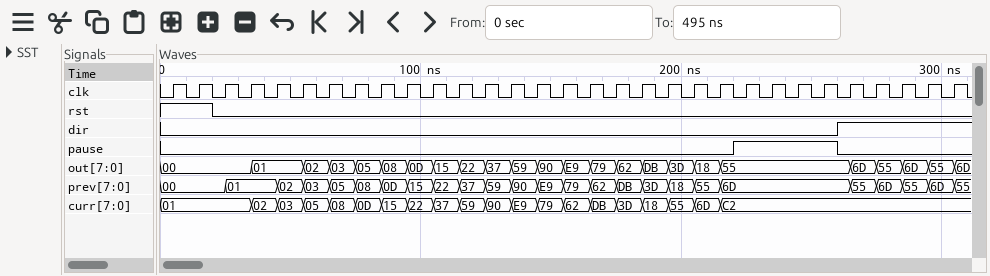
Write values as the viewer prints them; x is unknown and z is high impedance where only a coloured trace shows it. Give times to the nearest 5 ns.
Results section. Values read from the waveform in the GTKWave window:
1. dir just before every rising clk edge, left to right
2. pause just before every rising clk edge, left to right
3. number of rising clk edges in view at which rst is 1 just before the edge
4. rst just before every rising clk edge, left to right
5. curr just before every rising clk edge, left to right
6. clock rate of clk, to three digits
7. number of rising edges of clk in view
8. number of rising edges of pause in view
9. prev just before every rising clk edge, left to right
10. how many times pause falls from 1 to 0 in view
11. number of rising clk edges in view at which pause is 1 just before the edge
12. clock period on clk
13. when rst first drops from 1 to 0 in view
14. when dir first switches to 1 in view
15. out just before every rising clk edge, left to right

0 0 0 0 0 0 0 0 0 0 0 0 0 0 0 0 0 0 0 0 0 0 0 0 0 0 1 1 1 1 1
0 0 0 0 0 0 0 0 0 0 0 0 0 0 0 0 0 0 0 0 0 0 1 1 1 1 0 0 0 0 0
2
1 1 0 0 0 0 0 0 0 0 0 0 0 0 0 0 0 0 0 0 0 0 0 0 0 0 0 0 0 0 0
01, 01, 01, 01, 02, 03, 05, 08, 0D, 15, 22, 37, 59, 90, E9, 79, 62, DB, 3D, 18, 55, 6D, C2, C2, C2, C2, C2, C2, C2, C2, C2
100 MHz
31
1
00, 00, 00, 01, 01, 02, 03, 05, 08, 0D, 15, 22, 37, 59, 90, E9, 79, 62, DB, 3D, 18, 55, 6D, 6D, 6D, 6D, 6D, 55, 6D, 55, 6D
1
4
10 ns
20 ns
260 ns
00, 00, 00, 00, 01, 01, 02, 03, 05, 08, 0D, 15, 22, 37, 59, 90, E9, 79, 62, DB, 3D, 18, 55, 55, 55, 55, 55, 6D, 55, 6D, 55
